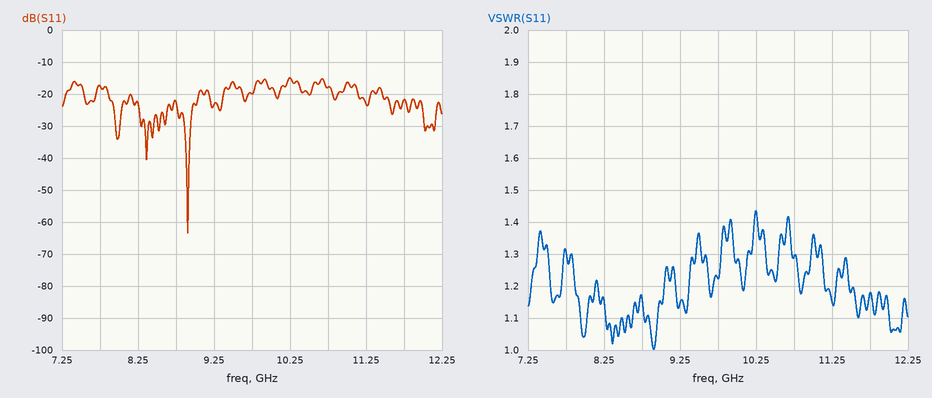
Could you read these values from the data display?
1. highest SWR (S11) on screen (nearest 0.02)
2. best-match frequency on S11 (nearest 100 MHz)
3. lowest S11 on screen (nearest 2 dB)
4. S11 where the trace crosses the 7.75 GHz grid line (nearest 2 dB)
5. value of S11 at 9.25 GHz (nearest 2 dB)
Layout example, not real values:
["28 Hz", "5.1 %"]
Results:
["1.44", "8.9 GHz", "-64 dB", "-18 dB", "-24 dB"]
